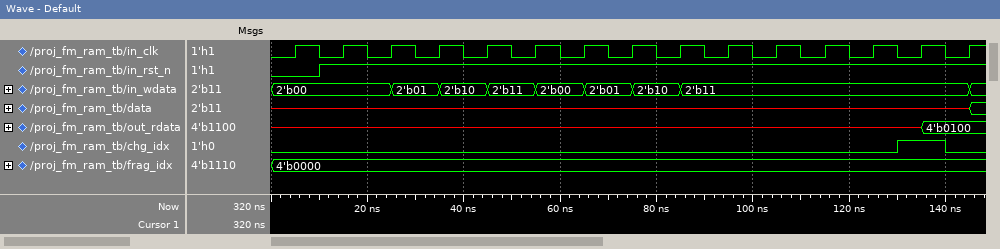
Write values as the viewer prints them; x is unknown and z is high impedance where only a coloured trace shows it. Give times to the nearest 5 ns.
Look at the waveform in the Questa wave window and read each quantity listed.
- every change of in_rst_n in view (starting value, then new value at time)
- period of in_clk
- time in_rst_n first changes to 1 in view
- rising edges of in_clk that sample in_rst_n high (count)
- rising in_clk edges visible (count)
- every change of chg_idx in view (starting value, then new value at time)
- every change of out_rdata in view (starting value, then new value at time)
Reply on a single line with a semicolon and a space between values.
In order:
0, 1 at 10 ns; 10 ns; 10 ns; 14; 15; 0, 1 at 130 ns, 0 at 140 ns; x, 4'b0100 at 135 ns
